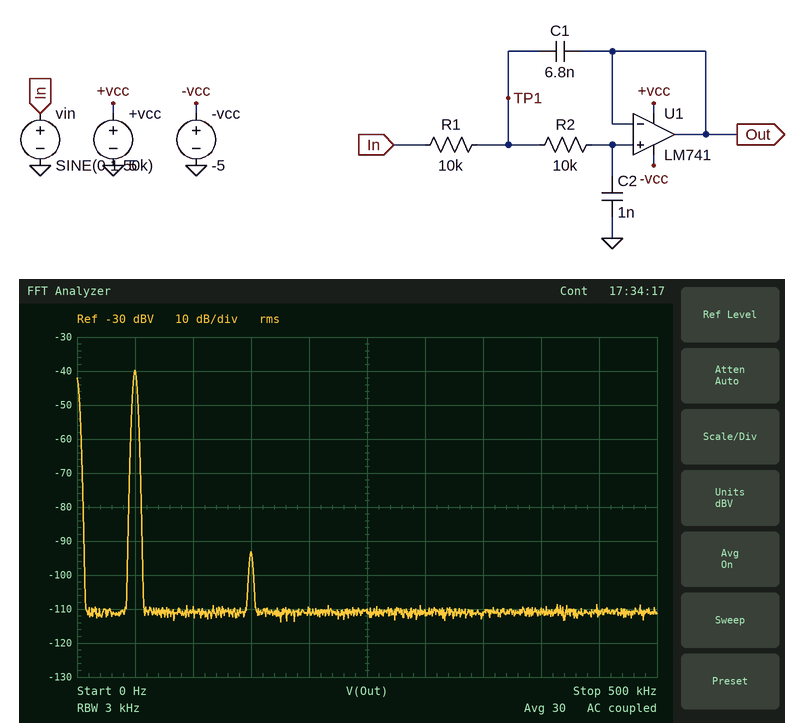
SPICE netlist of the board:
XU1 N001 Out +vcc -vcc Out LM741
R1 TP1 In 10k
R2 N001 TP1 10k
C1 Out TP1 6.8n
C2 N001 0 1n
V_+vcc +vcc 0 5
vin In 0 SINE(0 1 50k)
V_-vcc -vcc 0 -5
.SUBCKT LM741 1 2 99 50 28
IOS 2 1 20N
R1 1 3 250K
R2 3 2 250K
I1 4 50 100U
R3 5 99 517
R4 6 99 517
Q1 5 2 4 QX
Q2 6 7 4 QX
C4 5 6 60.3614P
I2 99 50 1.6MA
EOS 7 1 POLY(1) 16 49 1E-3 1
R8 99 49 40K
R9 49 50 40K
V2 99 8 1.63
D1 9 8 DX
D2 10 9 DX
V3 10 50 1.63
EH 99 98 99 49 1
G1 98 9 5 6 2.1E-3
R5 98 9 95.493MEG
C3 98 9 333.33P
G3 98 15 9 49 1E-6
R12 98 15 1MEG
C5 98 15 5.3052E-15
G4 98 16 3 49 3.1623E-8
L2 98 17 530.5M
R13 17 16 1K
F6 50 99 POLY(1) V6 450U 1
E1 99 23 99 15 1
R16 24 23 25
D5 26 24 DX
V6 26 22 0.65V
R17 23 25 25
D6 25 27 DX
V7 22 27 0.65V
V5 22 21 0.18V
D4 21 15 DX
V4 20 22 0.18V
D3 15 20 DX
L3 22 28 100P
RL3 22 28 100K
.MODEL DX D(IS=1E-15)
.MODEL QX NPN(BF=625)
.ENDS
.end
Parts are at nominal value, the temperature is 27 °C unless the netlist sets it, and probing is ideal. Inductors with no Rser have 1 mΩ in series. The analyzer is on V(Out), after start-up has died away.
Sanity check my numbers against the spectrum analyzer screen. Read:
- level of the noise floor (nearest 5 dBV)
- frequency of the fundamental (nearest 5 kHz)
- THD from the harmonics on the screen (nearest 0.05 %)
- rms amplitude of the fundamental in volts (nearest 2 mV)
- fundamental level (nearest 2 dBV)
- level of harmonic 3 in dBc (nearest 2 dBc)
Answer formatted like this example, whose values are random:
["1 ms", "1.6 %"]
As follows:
["-110 dBV", "50 kHz", "0.20 %", "10 mV", "-40 dBV", "-54 dBc"]
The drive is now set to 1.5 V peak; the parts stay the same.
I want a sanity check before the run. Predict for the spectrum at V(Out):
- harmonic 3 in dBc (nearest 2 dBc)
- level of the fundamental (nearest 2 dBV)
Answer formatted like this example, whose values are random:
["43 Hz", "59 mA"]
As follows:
["-48 dBc", "-36 dBV"]
